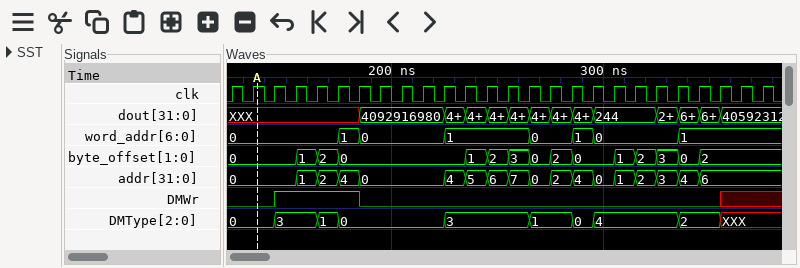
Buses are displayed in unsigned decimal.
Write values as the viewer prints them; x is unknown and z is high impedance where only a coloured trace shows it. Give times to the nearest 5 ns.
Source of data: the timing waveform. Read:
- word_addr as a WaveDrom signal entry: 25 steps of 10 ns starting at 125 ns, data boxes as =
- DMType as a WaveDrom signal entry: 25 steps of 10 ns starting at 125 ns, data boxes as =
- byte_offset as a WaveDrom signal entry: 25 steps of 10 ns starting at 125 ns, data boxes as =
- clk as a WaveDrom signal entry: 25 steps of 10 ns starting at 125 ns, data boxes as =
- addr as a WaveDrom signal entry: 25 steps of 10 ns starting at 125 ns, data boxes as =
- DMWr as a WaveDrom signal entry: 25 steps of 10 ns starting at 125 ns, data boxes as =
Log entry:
{name: 'word_addr', wave: '=....==...=...=.==...=...', data: '0 1 0 1 0 1 0 1'}
{name: 'DMType', wave: '=.=.==....=...=.==...=.x.', data: '0 3 1 0 3 1 0 4 2'}
{name: 'byte_offset', wave: '=..===.....======.=====..', data: '0 1 2 0 1 2 3 0 2 0 1 2 3 0 2'}
{name: 'clk', wave: 'p........................'}
{name: 'addr', wave: '=..====...=============..', data: '0 1 2 4 0 4 5 6 7 0 2 4 0 1 2 3 4 6'}
{name: 'DMWr', wave: '0.1...0................x.'}
